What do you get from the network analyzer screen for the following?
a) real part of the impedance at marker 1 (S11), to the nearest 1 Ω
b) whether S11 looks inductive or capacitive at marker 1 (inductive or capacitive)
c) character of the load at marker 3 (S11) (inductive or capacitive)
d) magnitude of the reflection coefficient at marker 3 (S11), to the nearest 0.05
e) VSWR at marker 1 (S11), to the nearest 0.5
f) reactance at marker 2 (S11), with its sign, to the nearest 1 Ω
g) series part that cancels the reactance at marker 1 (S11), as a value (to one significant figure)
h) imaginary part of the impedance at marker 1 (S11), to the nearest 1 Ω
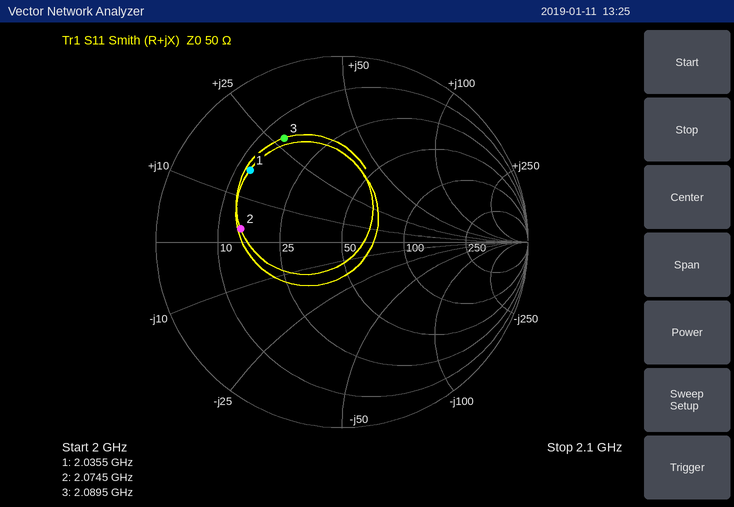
13 Ω
inductive
inductive
0.65
4.5
+3 Ω
5 pF
+16 Ω
